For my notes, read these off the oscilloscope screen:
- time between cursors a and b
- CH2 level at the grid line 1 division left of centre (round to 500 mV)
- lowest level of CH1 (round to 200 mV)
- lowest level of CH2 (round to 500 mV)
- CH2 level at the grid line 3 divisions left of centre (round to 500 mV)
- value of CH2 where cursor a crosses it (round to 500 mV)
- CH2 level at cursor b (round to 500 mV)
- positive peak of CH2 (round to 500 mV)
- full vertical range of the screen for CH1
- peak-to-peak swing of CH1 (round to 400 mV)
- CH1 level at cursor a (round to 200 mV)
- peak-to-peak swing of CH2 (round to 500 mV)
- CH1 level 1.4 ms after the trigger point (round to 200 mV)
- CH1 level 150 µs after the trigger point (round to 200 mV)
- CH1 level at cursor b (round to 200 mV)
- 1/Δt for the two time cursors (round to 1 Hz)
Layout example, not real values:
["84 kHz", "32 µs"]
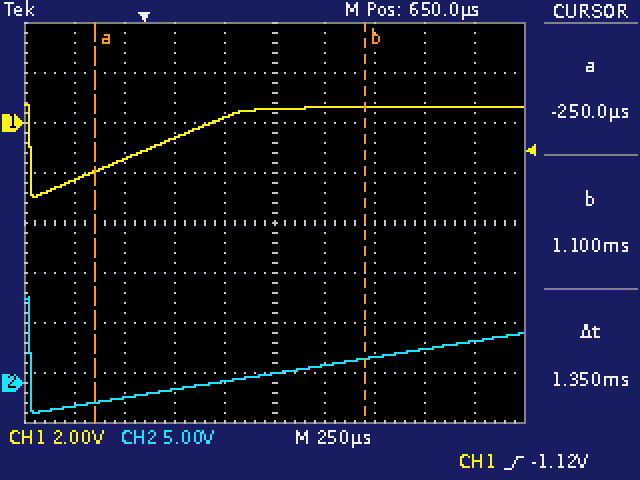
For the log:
["1.35 ms", "0.0 V", "-3.0 V", "-3.0 V", "-1.5 V", "-2.0 V", "2.5 V", "8.5 V", "16 V", "3.6 V", "-2.0 V", "11.5 V", "600 mV", "-600 mV", "600 mV", "741 Hz"]
